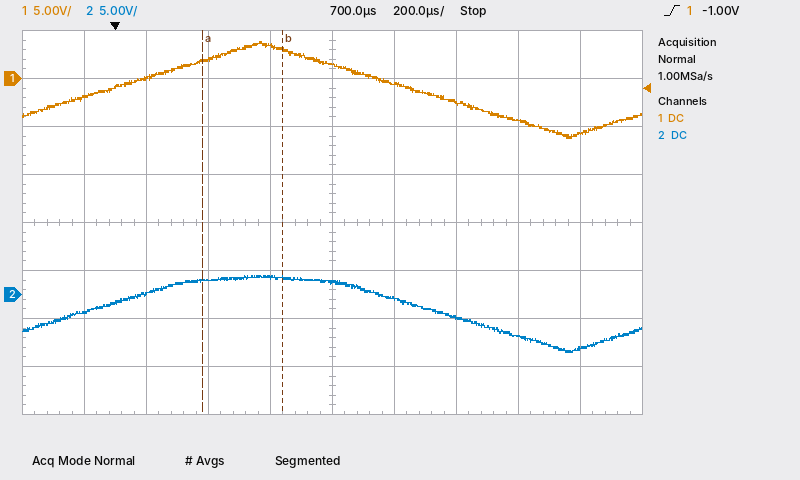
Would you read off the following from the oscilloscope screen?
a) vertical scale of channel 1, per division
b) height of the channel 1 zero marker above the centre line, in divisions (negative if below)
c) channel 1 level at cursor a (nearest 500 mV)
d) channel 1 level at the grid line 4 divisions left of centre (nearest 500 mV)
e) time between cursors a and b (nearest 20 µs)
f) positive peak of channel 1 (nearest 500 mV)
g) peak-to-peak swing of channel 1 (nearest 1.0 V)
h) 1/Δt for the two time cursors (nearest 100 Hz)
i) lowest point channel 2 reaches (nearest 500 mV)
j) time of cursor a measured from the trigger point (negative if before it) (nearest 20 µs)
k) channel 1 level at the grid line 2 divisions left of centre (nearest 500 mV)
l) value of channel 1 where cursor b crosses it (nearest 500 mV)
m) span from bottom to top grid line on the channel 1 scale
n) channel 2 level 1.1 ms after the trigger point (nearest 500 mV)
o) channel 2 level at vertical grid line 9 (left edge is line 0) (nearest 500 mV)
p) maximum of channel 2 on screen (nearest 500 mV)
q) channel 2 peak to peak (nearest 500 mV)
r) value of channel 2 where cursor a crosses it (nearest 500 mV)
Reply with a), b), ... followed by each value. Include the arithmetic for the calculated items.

a) 5 V
b) +3.0 div
c) 2.0 V
d) -2.0 V
e) 260 µs
f) 4.0 V
g) 10.0 V
h) 1 / 260 µs ≈ 3.8 kHz
i) -6.0 V
j) +280 µs
k) 2.0 V
l) 3.0 V
m) 40 V
n) -2.5 V
o) -5.5 V
p) 2.0 V
q) 2.0 V − (-6.0 V) = 8.0 V
r) 1.5 V
